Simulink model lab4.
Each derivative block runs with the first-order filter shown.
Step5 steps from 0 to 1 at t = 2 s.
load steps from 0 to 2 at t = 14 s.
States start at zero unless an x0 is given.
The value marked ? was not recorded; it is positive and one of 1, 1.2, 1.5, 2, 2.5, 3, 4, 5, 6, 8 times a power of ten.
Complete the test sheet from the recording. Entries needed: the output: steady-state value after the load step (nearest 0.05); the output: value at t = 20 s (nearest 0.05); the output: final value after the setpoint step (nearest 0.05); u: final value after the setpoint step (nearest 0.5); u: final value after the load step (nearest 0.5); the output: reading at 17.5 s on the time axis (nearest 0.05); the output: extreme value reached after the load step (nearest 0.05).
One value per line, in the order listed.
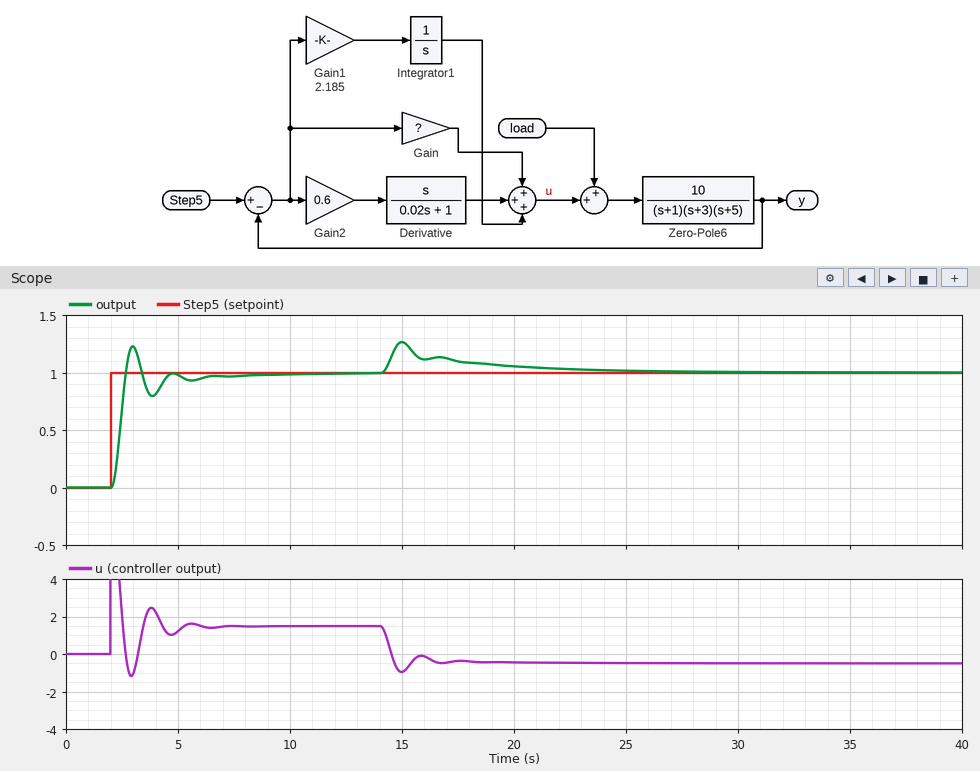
1.00
1.05
1.00
1.5
-0.5
1.10
1.25
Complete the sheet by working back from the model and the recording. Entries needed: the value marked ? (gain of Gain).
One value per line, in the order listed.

8
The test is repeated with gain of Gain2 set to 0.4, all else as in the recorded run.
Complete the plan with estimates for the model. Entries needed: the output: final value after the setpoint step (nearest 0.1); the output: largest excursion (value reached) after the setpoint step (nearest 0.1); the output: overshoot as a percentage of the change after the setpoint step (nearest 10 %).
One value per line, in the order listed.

1.0
1.3
30 %
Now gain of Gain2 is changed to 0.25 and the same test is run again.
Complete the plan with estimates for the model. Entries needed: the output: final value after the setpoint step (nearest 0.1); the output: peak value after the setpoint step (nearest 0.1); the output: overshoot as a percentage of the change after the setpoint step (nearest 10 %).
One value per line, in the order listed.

1.0
1.3
30 %
